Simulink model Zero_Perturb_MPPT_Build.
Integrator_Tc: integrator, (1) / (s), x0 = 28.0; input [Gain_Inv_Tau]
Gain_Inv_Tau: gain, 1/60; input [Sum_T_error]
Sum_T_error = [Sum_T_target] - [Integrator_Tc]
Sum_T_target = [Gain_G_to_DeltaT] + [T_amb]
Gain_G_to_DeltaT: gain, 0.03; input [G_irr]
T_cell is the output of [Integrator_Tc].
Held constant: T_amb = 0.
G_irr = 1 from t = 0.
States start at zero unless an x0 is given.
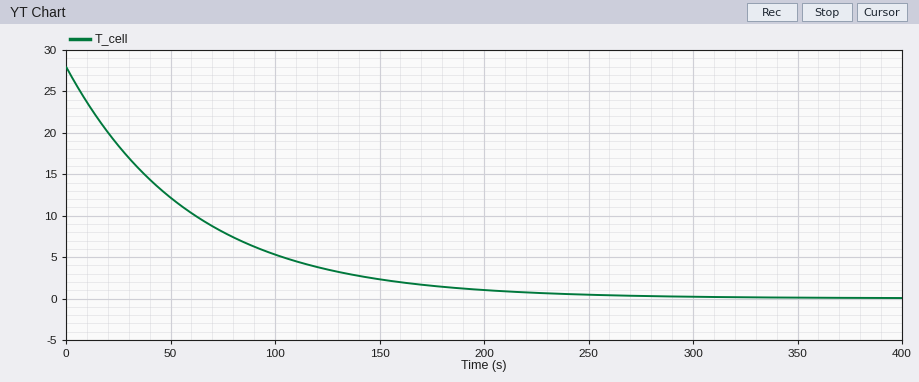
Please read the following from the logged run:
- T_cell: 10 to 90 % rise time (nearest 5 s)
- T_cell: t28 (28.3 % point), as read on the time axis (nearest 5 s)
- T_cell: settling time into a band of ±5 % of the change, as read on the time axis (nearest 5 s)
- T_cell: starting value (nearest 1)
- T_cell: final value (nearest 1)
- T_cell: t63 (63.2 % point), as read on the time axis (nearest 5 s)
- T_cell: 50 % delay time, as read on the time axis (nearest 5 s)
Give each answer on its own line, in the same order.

130 s
20 s
180 s
28
0
60 s
40 s
